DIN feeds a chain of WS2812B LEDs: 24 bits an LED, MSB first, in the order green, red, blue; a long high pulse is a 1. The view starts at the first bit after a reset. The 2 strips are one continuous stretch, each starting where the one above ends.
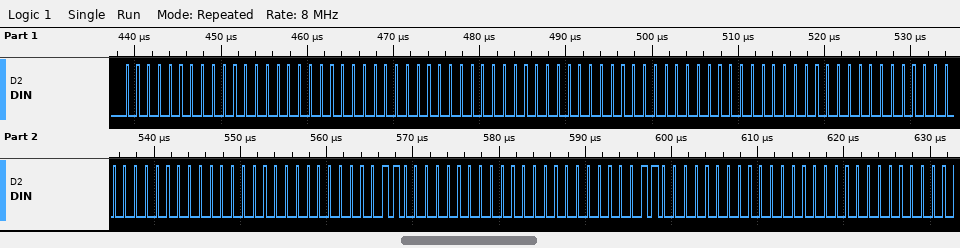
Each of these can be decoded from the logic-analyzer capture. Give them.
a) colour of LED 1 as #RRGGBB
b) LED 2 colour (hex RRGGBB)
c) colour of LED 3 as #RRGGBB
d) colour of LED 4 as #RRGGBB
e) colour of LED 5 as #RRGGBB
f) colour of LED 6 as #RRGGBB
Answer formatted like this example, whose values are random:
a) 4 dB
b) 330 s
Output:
a) #000000
b) #000000
c) #000000
d) #000000
e) #000300
f) #000300
